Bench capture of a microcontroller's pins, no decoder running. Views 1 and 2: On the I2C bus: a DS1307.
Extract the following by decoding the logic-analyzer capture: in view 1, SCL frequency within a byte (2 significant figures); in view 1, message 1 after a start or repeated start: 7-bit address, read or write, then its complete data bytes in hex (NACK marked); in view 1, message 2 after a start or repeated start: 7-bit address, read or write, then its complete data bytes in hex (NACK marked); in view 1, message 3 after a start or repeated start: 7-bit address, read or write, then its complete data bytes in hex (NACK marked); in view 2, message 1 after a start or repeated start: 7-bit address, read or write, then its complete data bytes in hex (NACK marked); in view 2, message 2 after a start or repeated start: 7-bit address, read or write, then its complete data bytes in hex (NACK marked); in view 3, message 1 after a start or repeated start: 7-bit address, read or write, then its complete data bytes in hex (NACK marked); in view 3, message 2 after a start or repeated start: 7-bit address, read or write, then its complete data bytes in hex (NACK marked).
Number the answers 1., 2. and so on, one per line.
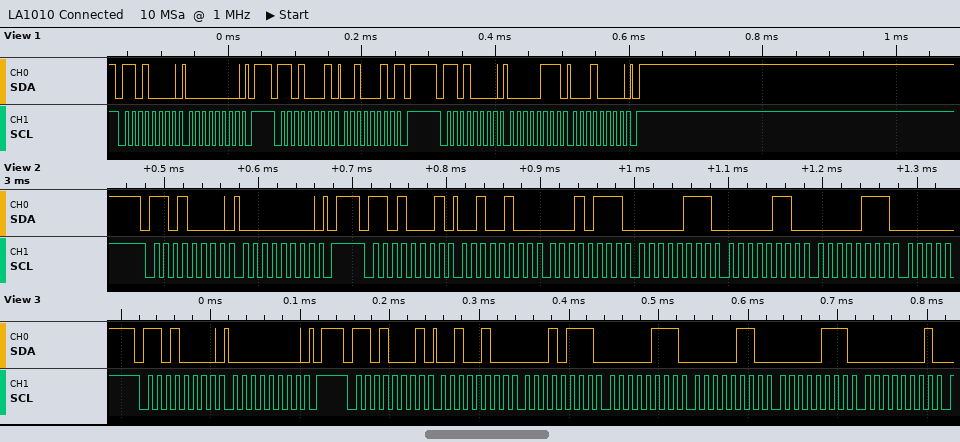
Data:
1. 100 kHz
2. 0x68 write: 00
3. 0x68 read: 22 NACK
4. 0x68 write: 07 10
5. 0x68 write: 00
6. 0x68 read: 24 17 07 06 07
7. 0x68 write: 00
8. 0x68 read: 24 17 07 06 07 01
